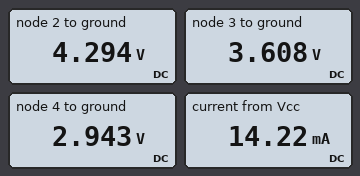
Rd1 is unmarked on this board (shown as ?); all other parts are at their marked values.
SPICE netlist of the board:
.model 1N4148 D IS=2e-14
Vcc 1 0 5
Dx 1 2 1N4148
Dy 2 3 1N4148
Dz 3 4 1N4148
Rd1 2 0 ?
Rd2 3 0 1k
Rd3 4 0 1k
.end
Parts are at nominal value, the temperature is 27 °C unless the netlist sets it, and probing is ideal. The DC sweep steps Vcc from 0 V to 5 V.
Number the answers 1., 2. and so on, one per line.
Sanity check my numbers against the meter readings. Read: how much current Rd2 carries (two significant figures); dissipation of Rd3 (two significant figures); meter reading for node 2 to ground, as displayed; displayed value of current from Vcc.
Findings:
1. 3.6 mA
2. 8.7 mW
3. 4.294 V
4. 14.22 mA
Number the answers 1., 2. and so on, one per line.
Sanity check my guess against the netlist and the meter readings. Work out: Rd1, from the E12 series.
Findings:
1. 560 Ω
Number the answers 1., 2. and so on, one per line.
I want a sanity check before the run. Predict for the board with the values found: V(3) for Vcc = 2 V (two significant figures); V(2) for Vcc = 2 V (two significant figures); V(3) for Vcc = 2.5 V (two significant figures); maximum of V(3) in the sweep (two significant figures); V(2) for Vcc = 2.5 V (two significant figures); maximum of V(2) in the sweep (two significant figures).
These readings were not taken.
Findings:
1. 700 mV
2. 1.3 V
3. 1.2 V
4. 3.6 V
5. 1.8 V
6. 4.3 V
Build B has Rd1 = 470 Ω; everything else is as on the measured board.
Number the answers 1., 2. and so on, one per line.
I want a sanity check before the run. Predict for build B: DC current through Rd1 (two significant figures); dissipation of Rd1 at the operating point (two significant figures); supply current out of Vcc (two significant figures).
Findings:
1. 9.1 mA
2. 39 mW
3. 16 mA
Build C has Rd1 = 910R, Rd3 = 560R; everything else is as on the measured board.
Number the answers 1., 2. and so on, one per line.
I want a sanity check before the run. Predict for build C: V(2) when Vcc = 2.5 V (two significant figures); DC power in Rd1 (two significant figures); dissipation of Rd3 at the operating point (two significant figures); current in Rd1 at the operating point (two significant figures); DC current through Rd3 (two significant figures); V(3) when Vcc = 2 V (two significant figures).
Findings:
1. 1.8 V
2. 20 mW
3. 15 mW
4. 4.7 mA
5. 5.2 mA
6. 710 mV
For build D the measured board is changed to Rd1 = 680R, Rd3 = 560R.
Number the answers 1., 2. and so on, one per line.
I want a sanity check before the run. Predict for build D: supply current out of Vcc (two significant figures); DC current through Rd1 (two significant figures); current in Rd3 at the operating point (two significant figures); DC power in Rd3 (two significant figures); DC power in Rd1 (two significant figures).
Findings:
1. 15 mA
2. 6.3 mA
3. 5.2 mA
4. 15 mW
5. 27 mW
